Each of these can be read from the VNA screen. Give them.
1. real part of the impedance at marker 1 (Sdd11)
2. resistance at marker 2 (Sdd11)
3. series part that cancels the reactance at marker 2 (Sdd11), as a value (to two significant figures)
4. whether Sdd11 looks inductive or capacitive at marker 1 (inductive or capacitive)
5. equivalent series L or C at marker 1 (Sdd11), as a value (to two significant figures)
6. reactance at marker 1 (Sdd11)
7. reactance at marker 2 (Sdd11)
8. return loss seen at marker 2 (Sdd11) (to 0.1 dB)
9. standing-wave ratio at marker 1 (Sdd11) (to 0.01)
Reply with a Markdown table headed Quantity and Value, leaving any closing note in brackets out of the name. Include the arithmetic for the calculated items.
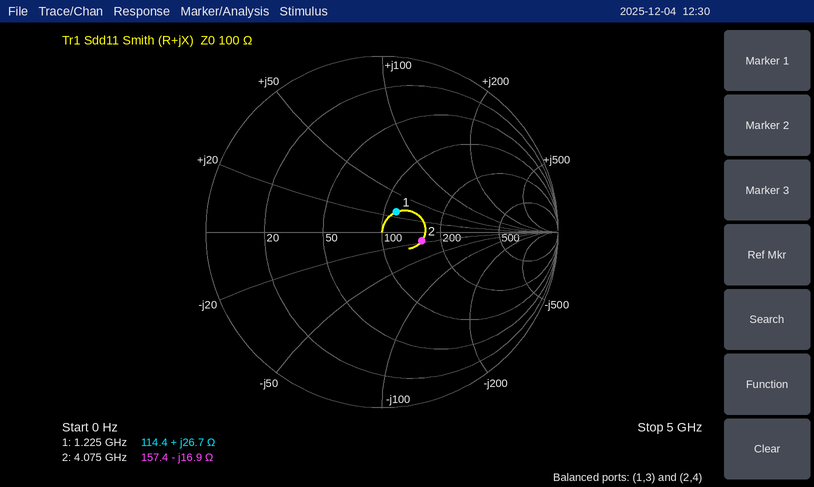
| Quantity | Value |
|---|---|
| real part of the impedance at marker 1 | 114.4 Ω |
| resistance at marker 2 | 157.4 Ω |
| series part that cancels the reactance at marker 2 (Sdd11), as a value | L = 16.9 Ω/(2π × 4.075 GHz) ≈ 660 pH |
| whether Sdd11 looks inductive or capacitive at marker 1 | inductive |
| equivalent series L or C at marker 1 (Sdd11), as a value | L = 26.7 Ω/(2π × 1.225 GHz) ≈ 3.5 nH |
| reactance at marker 1 | +26.7 Ω |
| reactance at marker 2 | -16.9 Ω |
| return loss seen at marker 2 (Sdd11) | 12.7 dB |
| standing-wave ratio at marker 1 (Sdd11) | 1.33 |
